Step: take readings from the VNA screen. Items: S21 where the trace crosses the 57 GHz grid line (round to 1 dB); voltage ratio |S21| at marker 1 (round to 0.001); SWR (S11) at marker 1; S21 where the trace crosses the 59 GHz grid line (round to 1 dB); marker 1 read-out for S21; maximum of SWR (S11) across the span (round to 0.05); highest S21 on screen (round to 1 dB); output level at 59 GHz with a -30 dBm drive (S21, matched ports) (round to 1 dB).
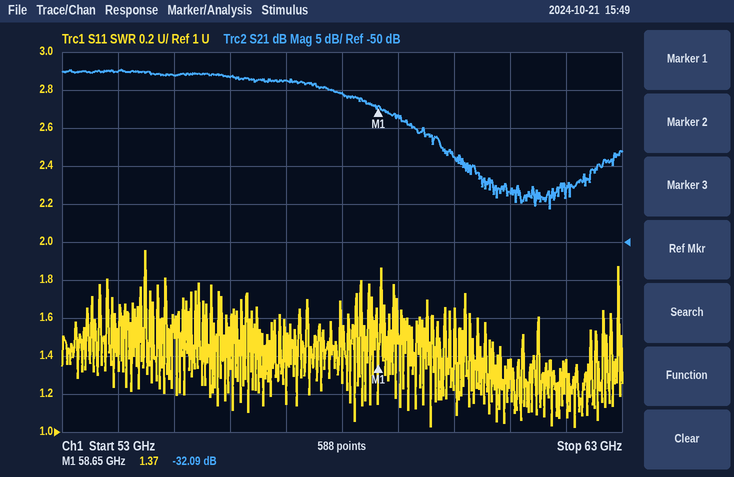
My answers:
-29 dB
0.025
1.37
-33 dB
-32.09 dB
1.95
-27 dB
-63 dBm
